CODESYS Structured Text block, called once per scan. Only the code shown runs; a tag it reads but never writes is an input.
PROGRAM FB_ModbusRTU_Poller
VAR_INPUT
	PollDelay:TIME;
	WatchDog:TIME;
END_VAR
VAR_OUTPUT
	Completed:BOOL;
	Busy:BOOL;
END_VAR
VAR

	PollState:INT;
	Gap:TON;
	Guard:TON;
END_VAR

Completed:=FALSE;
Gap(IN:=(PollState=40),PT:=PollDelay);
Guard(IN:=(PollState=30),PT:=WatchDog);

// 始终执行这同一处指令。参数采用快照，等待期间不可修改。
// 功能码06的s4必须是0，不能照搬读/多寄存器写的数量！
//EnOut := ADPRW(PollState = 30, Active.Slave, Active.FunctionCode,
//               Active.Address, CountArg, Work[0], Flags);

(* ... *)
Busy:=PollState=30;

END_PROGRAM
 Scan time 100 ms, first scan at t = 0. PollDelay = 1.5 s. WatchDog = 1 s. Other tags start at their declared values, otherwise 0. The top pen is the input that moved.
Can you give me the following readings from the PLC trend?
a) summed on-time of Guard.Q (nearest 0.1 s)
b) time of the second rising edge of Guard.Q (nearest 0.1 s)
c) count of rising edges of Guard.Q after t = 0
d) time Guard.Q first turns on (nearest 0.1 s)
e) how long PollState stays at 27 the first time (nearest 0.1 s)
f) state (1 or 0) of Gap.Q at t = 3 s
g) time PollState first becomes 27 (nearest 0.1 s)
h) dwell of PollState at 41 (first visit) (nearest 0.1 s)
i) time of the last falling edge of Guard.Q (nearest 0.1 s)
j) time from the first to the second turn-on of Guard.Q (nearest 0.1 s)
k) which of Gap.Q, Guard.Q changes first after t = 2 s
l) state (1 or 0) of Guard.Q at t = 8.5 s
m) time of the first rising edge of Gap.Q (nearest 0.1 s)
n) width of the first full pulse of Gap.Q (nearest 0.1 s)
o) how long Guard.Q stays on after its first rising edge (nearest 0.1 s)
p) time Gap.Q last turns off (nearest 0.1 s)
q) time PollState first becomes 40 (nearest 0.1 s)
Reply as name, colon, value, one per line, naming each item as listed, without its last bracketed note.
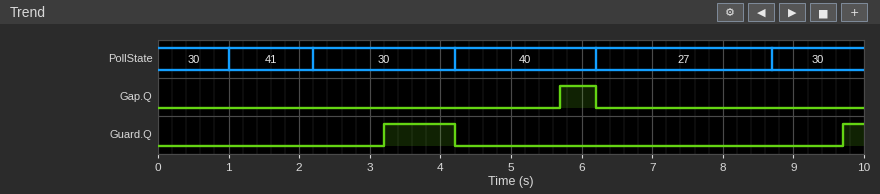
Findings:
summed on-time of Guard.Q: 1.3 s
time of the second rising edge of Guard.Q: 9.7 s
count of rising edges of Guard.Q after t = 0: 2
time Guard.Q first turns on: 3.2 s
how long PollState stays at 27 the first time: 2.5 s
state (1 or 0) of Gap.Q at t = 3 s: 0
time PollState first becomes 27: 6.2 s
dwell of PollState at 41 (first visit): 1.2 s
time of the last falling edge of Guard.Q: 4.2 s
time from the first to the second turn-on of Guard.Q: 6.5 s
which of Gap.Q, Guard.Q changes first after t = 2 s: Guard.Q
state (1 or 0) of Guard.Q at t = 8.5 s: 0
time of the first rising edge of Gap.Q: 5.7 s
width of the first full pulse of Gap.Q: 0.5 s
how long Guard.Q stays on after its first rising edge: 1.0 s
time Gap.Q last turns off: 6.2 s
time PollState first becomes 40: 4.2 s
